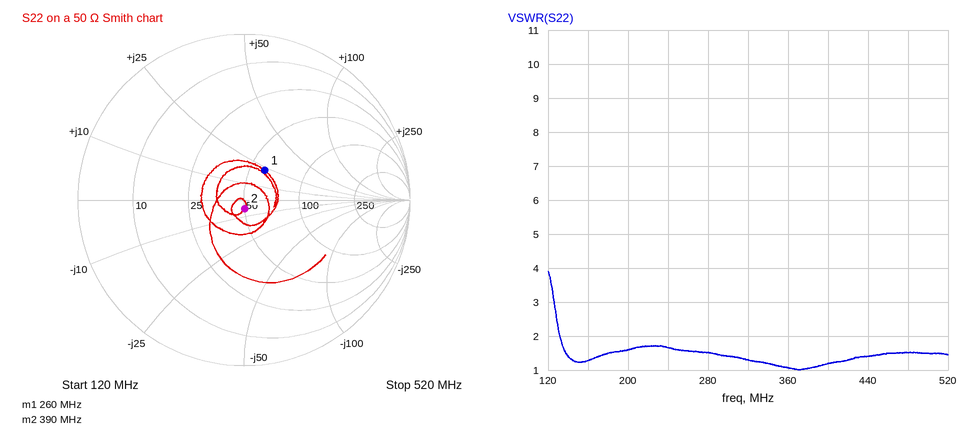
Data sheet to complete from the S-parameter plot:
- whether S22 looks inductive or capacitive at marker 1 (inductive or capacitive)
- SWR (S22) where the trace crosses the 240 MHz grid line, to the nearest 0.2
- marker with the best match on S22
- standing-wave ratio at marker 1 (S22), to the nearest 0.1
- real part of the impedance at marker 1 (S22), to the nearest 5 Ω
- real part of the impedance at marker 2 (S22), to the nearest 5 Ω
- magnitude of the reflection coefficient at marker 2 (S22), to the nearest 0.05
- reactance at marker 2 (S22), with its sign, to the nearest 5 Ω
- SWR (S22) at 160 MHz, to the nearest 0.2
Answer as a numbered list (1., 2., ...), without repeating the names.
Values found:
1. inductive
2. 1.6
3. marker 2
4. 1.6
5. 60 Ω
6. 50 Ω
7. 0.05
8. -5 Ω
9. 1.2
